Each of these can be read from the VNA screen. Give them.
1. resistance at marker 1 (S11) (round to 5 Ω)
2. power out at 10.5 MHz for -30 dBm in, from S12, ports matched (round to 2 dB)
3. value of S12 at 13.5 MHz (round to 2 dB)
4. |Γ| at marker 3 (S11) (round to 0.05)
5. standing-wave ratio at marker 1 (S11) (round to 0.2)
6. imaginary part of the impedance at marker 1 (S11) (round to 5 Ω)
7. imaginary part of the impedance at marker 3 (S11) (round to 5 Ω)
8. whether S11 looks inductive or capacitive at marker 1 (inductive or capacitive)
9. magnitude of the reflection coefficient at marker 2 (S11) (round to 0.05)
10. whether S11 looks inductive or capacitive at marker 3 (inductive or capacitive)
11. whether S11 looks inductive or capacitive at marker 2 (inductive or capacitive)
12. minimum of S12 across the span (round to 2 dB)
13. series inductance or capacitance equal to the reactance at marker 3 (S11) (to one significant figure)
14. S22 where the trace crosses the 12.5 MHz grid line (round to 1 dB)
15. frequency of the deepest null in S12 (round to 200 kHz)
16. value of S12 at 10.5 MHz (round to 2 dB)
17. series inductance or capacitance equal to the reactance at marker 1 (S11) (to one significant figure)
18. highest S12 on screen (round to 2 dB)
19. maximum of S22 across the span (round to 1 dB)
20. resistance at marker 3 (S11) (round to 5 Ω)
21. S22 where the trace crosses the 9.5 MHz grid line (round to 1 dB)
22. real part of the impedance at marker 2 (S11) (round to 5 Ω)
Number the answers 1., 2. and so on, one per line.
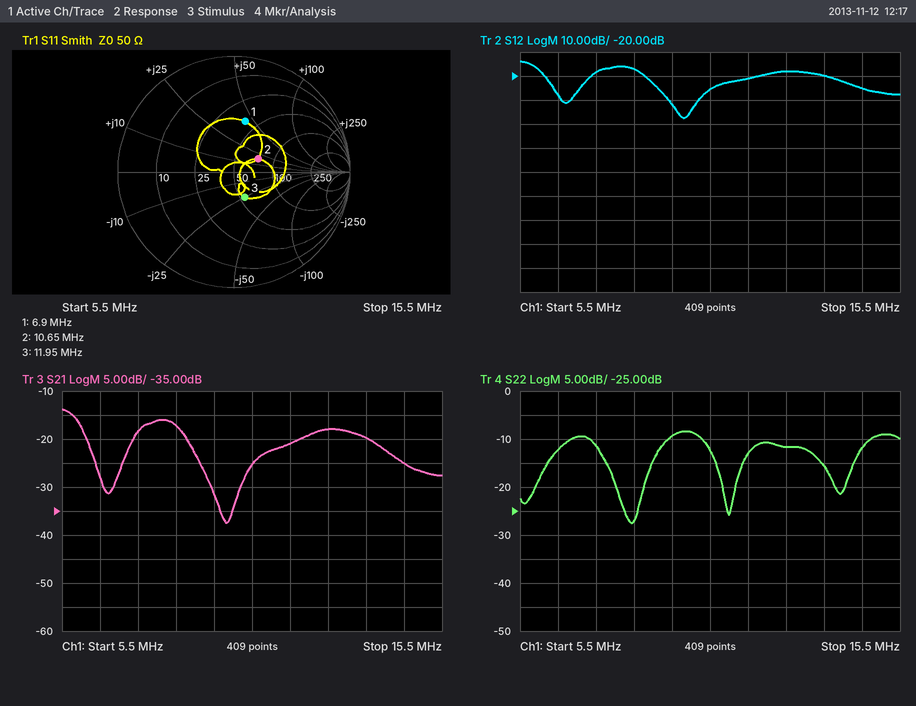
1. 40 Ω
2. -56 dBm
3. -20 dB
4. 0.25
5. 2.6
6. +45 Ω
7. -25 Ω
8. inductive
9. 0.25
10. capacitive
11. inductive
12. -38 dB
13. 500 pF
14. -12 dB
15. 9.8 MHz
16. -26 dB
17. 1.0 µH
18. -14 dB
19. -8 dB
20. 55 Ω
21. -9 dB
22. 75 Ω
